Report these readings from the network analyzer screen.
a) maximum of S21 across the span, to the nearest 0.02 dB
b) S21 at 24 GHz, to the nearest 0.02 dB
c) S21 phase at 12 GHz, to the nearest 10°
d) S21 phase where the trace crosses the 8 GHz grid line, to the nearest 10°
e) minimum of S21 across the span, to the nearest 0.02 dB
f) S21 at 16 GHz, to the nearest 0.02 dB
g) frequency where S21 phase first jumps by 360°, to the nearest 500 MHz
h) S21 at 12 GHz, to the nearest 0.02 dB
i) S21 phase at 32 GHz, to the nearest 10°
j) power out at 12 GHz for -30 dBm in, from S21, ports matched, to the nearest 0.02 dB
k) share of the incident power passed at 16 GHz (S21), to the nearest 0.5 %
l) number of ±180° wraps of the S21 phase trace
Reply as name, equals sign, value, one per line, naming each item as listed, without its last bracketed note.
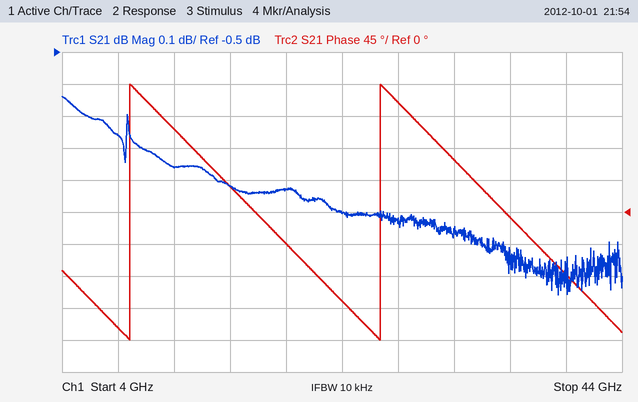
maximum of S21 across the span, to the nearest 0.02 dB = -0.64 dB
S21 at 24 GHz, to the nearest 0.02 dB = -1.00 dB
S21 phase at 12 GHz, to the nearest 10° = 120°
S21 phase where the trace crosses the 8 GHz grid line, to the nearest 10° = -160°
minimum of S21 across the span, to the nearest 0.02 dB = -1.26 dB
S21 at 16 GHz, to the nearest 0.02 dB = -0.92 dB
frequency where S21 phase first jumps by 360°, to the nearest 500 MHz = 9.0 GHz
S21 at 12 GHz, to the nearest 0.02 dB = -0.86 dB
S21 phase at 32 GHz, to the nearest 10° = 70°
power out at 12 GHz for -30 dBm in, from S21, ports matched, to the nearest 0.02 dB = -30.86 dBm
share of the incident power passed at 16 GHz (S21), to the nearest 0.5 % = 81.0 %
number of ±180° wraps of the S21 phase trace = 2
